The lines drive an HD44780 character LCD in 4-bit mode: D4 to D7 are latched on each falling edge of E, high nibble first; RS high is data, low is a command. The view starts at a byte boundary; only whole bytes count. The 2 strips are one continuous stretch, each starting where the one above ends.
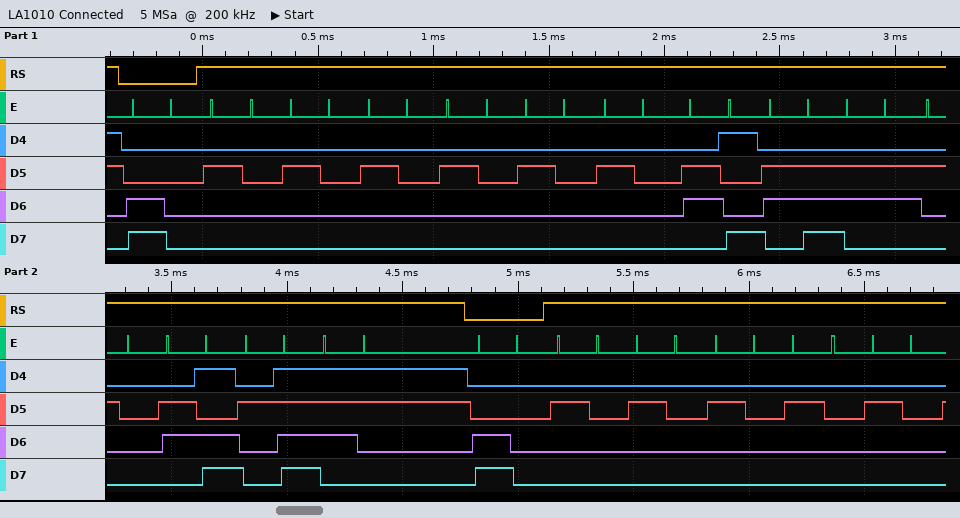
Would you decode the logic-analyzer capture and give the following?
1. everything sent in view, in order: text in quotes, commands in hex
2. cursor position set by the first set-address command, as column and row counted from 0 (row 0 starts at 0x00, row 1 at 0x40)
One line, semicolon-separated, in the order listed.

0xC0 "      inf m/s" 0xC0 "     "; column 0, row 1
